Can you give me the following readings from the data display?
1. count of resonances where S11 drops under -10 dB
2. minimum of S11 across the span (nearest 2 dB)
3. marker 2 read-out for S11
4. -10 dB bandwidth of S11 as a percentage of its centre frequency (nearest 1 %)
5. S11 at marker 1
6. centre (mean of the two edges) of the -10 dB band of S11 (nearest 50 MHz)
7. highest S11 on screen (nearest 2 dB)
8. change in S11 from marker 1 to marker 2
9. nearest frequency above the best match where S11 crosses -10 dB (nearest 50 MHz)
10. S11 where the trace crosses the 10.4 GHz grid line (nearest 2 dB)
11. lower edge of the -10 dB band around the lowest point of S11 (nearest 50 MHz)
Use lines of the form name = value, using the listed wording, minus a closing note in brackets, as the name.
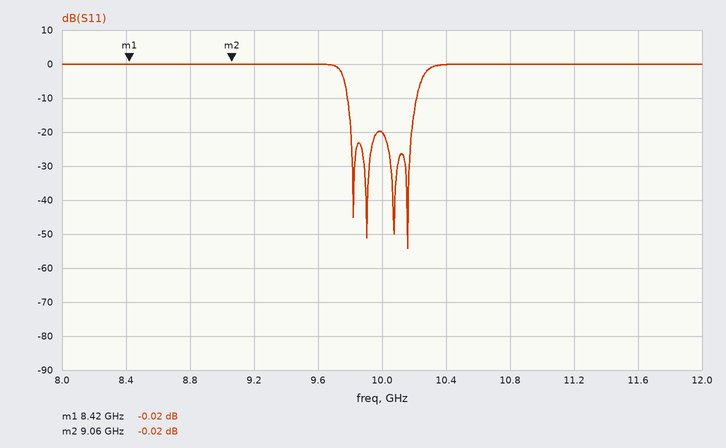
count of resonances where S11 drops under -10 dB = 4
minimum of S11 across the span = -54 dB
marker 2 read-out for S11 = -0.02 dB
-10 dB bandwidth of S11 as a percentage of its centre frequency = 4 %
S11 at marker 1 = -0.02 dB
centre (mean of the two edges) of the -10 dB band of S11 = 10.00 GHz
highest S11 on screen = 0 dB
change in S11 from marker 1 to marker 2 = 0.00 dB
nearest frequency above the best match where S11 crosses -10 dB = 10.20 GHz
S11 where the trace crosses the 10.4 GHz grid line = 0 dB
lower edge of the -10 dB band around the lowest point of S11 = 9.80 GHz
